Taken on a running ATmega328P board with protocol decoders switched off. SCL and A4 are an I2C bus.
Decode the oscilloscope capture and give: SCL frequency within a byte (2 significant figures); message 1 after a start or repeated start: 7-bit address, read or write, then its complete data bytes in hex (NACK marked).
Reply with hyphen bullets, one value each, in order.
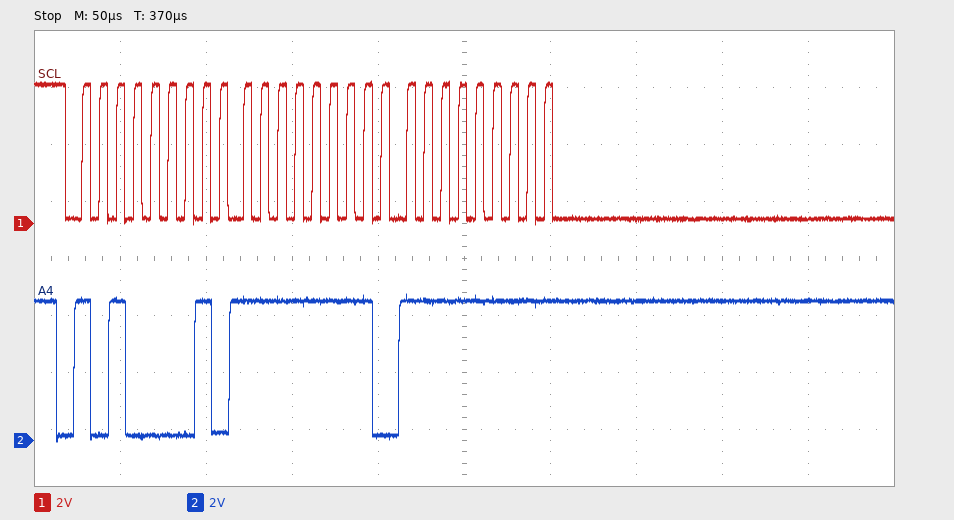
- 100 kHz
- 0x50 read: FF FF NACK
